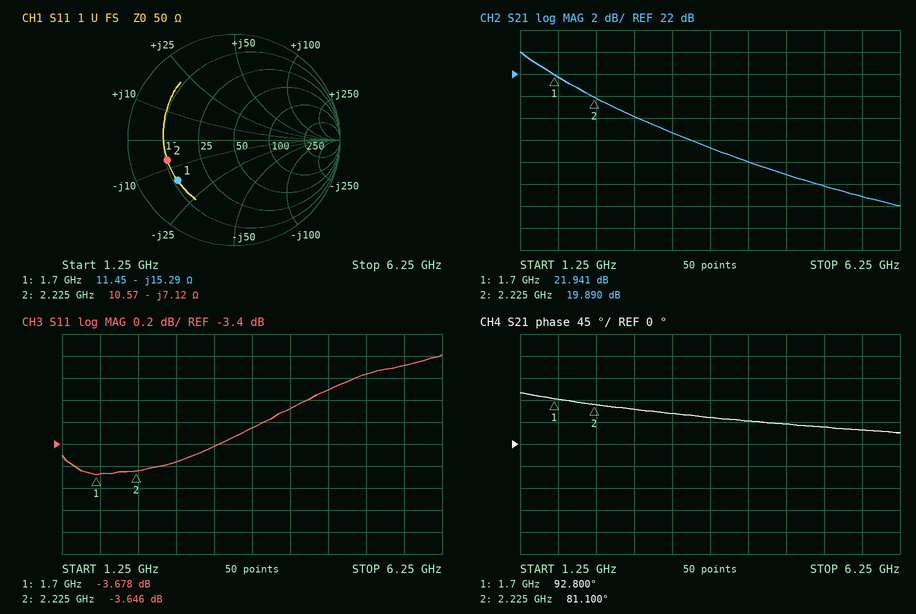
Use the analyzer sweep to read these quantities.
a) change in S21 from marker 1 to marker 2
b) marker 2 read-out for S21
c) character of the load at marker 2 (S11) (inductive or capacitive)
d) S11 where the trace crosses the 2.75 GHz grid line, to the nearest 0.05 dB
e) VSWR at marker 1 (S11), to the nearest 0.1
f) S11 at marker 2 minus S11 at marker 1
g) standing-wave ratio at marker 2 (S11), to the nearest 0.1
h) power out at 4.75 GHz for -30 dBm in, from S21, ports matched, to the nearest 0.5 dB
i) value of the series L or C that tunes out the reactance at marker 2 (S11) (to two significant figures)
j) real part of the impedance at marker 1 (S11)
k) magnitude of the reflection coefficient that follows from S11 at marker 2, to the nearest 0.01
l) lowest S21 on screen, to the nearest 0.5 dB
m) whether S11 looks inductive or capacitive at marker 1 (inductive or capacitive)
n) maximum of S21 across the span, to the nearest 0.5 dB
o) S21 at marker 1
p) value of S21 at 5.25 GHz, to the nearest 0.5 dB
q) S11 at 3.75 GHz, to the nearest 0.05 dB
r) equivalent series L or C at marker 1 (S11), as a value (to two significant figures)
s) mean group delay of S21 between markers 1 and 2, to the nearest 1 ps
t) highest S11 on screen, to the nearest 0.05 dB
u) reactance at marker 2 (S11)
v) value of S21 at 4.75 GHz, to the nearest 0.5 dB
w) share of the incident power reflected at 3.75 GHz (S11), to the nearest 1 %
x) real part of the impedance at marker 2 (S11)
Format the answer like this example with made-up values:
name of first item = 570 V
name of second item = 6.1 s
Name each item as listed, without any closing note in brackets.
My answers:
change in S21 from marker 1 to marker 2 = -2.051 dB
marker 2 read-out for S21 = 19.890 dB
character of the load at marker 2 (S11) = capacitive
S11 where the trace crosses the 2.75 GHz grid line, to the nearest 0.05 dB = -3.55 dB
VSWR at marker 1 (S11), to the nearest 0.1 = 4.8
S11 at marker 2 minus S11 at marker 1 = 0.032 dB
standing-wave ratio at marker 2 (S11), to the nearest 0.1 = 4.8
power out at 4.75 GHz for -30 dBm in, from S21, ports matched, to the nearest 0.5 dB = -17.0 dBm
value of the series L or C that tunes out the reactance at marker 2 (S11) = 510 pH
real part of the impedance at marker 1 = 11.45 Ω
magnitude of the reflection coefficient that follows from S11 at marker 2, to the nearest 0.01 = 0.66
lowest S21 on screen, to the nearest 0.5 dB = 10.0 dB
whether S11 looks inductive or capacitive at marker 1 = capacitive
maximum of S21 across the span, to the nearest 0.5 dB = 24.0 dB
S21 at marker 1 = 21.941 dB
value of S21 at 5.25 GHz, to the nearest 0.5 dB = 12.0 dB
S11 at 3.75 GHz, to the nearest 0.05 dB = -3.25 dB
equivalent series L or C at marker 1 (S11), as a value = 6.1 pF
mean group delay of S21 between markers 1 and 2, to the nearest 1 ps = 62 ps
highest S11 on screen, to the nearest 0.05 dB = -2.60 dB
reactance at marker 2 = -7.12 Ω
value of S21 at 4.75 GHz, to the nearest 0.5 dB = 13.0 dB
share of the incident power reflected at 3.75 GHz (S11), to the nearest 1 % = 47 %
real part of the impedance at marker 2 = 10.57 Ω
